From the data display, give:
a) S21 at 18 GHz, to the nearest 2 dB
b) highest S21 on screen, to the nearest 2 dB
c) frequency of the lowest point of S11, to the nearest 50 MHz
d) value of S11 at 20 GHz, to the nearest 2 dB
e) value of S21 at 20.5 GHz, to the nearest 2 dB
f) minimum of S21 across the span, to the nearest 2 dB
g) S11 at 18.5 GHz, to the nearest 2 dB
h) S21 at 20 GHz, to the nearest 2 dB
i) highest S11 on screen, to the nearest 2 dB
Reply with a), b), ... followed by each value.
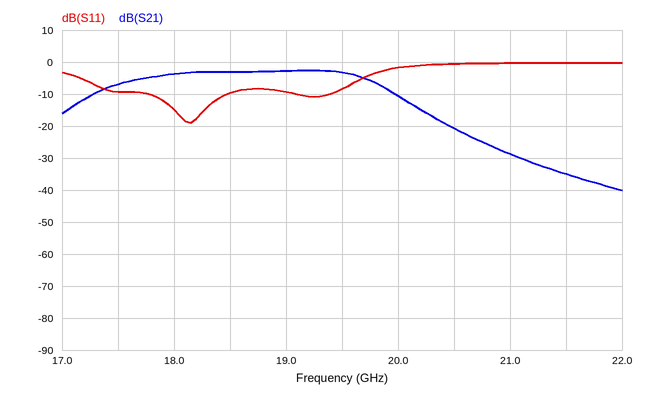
a) -4 dB
b) -2 dB
c) 18.15 GHz
d) -2 dB
e) -20 dB
f) -40 dB
g) -10 dB
h) -10 dB
i) 0 dB
